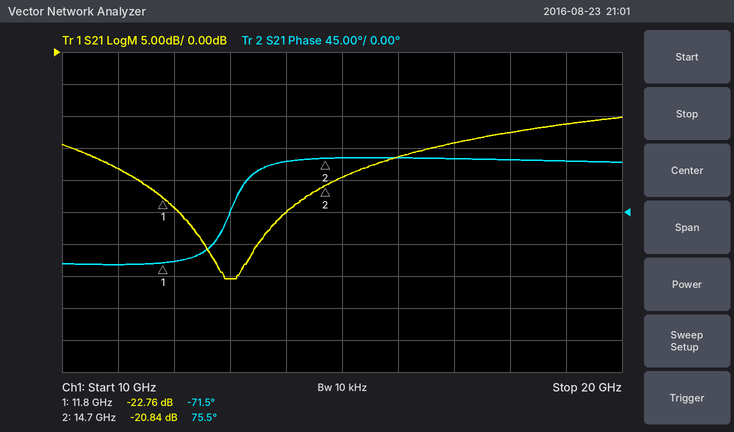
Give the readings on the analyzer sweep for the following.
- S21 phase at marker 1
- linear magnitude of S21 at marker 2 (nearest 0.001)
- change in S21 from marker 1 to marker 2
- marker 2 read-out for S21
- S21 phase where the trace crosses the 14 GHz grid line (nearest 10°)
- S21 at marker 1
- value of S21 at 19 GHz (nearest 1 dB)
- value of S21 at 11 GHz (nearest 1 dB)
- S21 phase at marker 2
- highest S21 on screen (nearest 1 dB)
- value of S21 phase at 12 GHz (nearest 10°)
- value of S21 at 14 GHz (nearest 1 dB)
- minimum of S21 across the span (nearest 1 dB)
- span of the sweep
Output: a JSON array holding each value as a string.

["-71.5°", "0.091", "1.92 dB", "-20.84 dB", "70°", "-22.76 dB", "-11 dB", "-18 dB", "75.5°", "-10 dB", "-70°", "-25 dB", "-35 dB", "10 GHz"]
